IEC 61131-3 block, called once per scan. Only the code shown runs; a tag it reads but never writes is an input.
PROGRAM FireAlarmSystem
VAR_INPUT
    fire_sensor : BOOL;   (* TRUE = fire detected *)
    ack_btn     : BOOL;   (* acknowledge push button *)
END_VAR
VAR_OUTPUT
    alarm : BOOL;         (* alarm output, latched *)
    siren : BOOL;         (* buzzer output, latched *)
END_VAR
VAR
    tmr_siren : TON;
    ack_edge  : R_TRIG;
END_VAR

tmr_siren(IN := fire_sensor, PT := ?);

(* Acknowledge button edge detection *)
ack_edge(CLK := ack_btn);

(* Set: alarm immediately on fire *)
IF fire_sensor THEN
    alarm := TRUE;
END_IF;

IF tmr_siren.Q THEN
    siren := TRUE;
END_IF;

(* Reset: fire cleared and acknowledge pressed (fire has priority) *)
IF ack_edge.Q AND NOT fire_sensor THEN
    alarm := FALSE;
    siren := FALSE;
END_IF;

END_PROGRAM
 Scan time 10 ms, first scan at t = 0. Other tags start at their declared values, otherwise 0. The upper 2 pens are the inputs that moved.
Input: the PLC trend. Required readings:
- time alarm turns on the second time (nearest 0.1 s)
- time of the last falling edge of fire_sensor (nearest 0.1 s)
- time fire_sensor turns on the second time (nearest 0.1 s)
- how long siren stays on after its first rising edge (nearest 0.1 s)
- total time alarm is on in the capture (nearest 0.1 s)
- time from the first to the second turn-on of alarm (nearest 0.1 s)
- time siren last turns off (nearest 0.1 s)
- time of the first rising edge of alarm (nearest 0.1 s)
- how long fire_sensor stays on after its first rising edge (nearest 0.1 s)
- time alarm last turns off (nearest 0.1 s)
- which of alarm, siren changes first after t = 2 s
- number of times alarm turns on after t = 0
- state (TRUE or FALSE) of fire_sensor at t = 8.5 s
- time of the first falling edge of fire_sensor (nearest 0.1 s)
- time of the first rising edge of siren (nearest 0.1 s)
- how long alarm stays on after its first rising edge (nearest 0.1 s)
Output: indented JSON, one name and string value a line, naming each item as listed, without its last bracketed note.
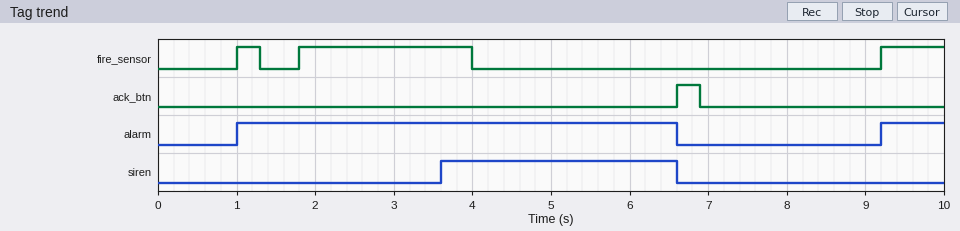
{
  "time alarm turns on the second time": "9.2 s",
  "time of the last falling edge of fire_sensor": "4.0 s",
  "time fire_sensor turns on the second time": "1.8 s",
  "how long siren stays on after its first rising edge": "3.0 s",
  "total time alarm is on in the capture": "6.4 s",
  "time from the first to the second turn-on of alarm": "8.2 s",
  "time siren last turns off": "6.6 s",
  "time of the first rising edge of alarm": "1.0 s",
  "how long fire_sensor stays on after its first rising edge": "0.3 s",
  "time alarm last turns off": "6.6 s",
  "which of alarm, siren changes first after t = 2 s": "siren",
  "number of times alarm turns on after t = 0": "2",
  "state (TRUE or FALSE) of fire_sensor at t = 8.5 s": "FALSE",
  "time of the first falling edge of fire_sensor": "1.3 s",
  "time of the first rising edge of siren": "3.6 s",
  "how long alarm stays on after its first rising edge": "5.6 s"
}
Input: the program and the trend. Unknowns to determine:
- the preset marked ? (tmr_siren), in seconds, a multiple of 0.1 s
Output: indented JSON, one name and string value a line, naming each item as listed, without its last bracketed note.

{
  "the preset marked ? (tmr_siren), in seconds, a multiple of 0.1 s": "1.8 s"
}
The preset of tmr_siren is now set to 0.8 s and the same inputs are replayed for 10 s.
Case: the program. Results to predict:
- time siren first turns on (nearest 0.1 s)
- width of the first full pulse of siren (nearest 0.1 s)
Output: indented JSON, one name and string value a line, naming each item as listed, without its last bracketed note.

{
  "time siren first turns on": "2.6 s",
  "width of the first full pulse of siren": "4.0 s"
}
